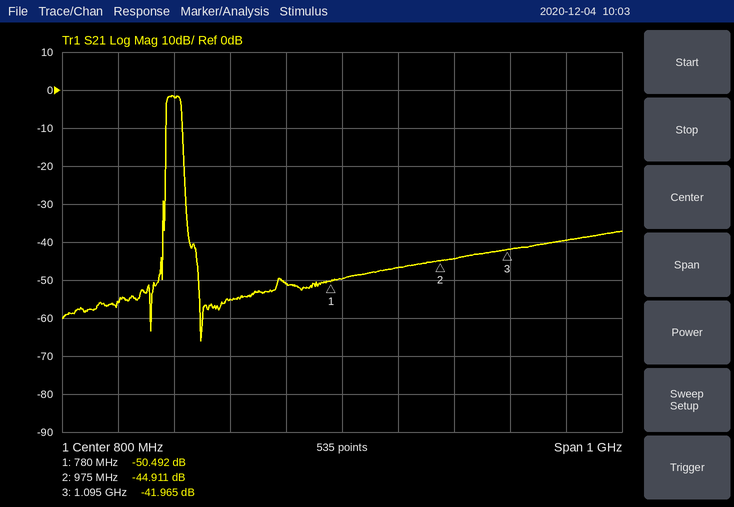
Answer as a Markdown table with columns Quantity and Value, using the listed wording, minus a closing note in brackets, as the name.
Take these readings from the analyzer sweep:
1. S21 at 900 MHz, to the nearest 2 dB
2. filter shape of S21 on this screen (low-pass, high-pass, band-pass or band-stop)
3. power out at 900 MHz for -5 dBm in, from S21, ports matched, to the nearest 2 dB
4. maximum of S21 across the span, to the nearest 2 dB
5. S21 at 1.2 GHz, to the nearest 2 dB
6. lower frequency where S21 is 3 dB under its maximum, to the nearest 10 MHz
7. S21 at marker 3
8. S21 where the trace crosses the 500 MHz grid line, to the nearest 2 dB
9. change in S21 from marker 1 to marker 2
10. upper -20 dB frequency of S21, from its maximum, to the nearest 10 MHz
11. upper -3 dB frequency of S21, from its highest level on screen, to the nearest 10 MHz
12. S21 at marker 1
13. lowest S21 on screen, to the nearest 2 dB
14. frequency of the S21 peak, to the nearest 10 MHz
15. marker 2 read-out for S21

| Quantity | Value |
|---|---|
| S21 at 900 MHz, to the nearest 2 dB | -46 dB |
| filter shape of S21 on this screen | band-pass |
| power out at 900 MHz for -5 dBm in, from S21, ports matched, to the nearest 2 dB | -52 dBm |
| maximum of S21 across the span, to the nearest 2 dB | -2 dB |
| S21 at 1.2 GHz, to the nearest 2 dB | -40 dB |
| lower frequency where S21 is 3 dB under its maximum, to the nearest 10 MHz | 490 MHz |
| S21 at marker 3 | -41.965 dB |
| S21 where the trace crosses the 500 MHz grid line, to the nearest 2 dB | -2 dB |
| change in S21 from marker 1 to marker 2 | 5.581 dB |
| upper -20 dB frequency of S21, from its maximum, to the nearest 10 MHz | 520 MHz |
| upper -3 dB frequency of S21, from its highest level on screen, to the nearest 10 MHz | 510 MHz |
| S21 at marker 1 | -50.492 dB |
| lowest S21 on screen, to the nearest 2 dB | -66 dB |
| frequency of the S21 peak, to the nearest 10 MHz | 500 MHz |
| marker 2 read-out for S21 | -44.911 dB |
